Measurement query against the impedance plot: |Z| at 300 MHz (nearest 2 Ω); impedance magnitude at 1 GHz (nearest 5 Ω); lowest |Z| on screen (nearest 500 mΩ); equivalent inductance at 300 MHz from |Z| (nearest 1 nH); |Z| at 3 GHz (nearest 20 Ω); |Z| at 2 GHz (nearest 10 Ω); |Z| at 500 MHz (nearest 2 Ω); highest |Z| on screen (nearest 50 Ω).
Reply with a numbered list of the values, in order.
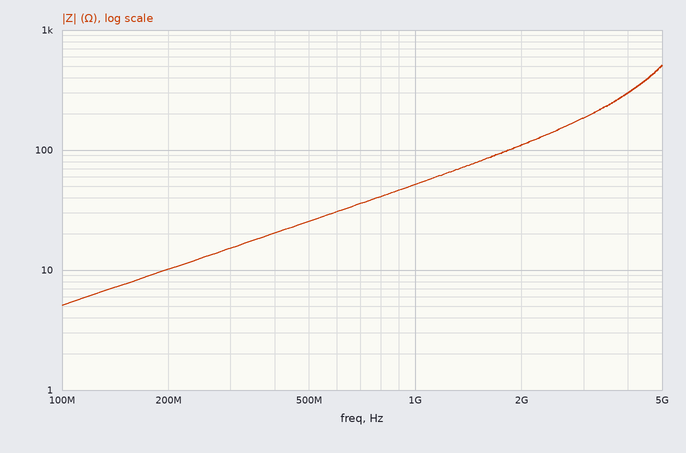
1. 16 Ω
2. 50 Ω
3. 5.0 Ω
4. 8 nH
5. 180 Ω
6. 110 Ω
7. 26 Ω
8. 500 Ω
